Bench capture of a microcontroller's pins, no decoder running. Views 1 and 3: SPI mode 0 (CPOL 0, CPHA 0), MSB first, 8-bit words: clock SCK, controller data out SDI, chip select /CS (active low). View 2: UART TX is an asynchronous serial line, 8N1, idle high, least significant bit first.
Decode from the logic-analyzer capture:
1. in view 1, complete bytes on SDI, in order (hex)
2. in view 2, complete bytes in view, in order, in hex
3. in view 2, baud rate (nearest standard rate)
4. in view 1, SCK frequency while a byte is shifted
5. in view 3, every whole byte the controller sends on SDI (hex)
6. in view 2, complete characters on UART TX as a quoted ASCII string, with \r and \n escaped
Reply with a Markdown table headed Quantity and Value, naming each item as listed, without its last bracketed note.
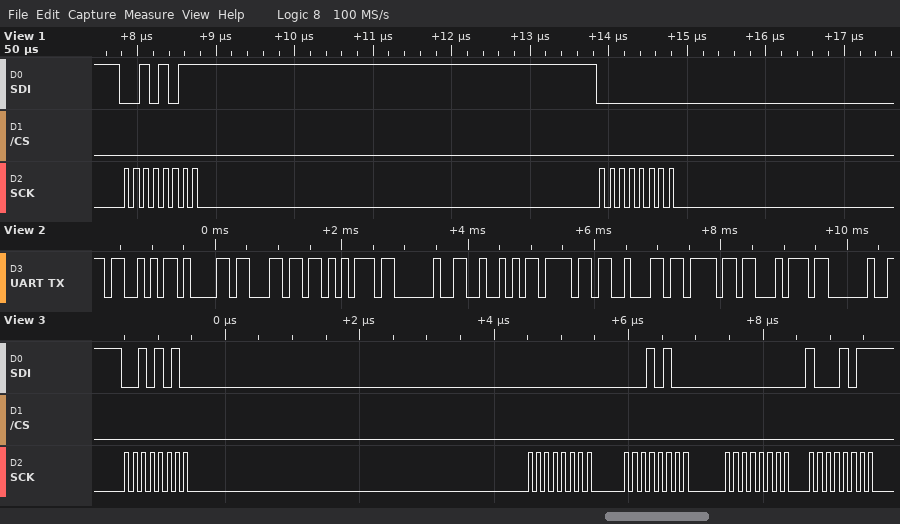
| Quantity | Value |
|---|---|
| in view 1, complete bytes on SDI, in order | 0x2B 0x00 |
| in view 2, complete bytes in view, in order, in hex | 0x53 0x61 0x6C 0x75 0x20 0x52 0x6F 0x62 0x6F 0x74 0x20 |
| in view 2, baud rate | 9600 baud |
| in view 1, SCK frequency while a byte is shifted | 8 MHz |
| in view 3, every whole byte the controller sends on SDI | 0x2A 0x00 0x14 0x00 0x8B |
| in view 2, complete characters on UART TX as a quoted ASCII string, with \r and \n escaped | "Salu Robot " |
